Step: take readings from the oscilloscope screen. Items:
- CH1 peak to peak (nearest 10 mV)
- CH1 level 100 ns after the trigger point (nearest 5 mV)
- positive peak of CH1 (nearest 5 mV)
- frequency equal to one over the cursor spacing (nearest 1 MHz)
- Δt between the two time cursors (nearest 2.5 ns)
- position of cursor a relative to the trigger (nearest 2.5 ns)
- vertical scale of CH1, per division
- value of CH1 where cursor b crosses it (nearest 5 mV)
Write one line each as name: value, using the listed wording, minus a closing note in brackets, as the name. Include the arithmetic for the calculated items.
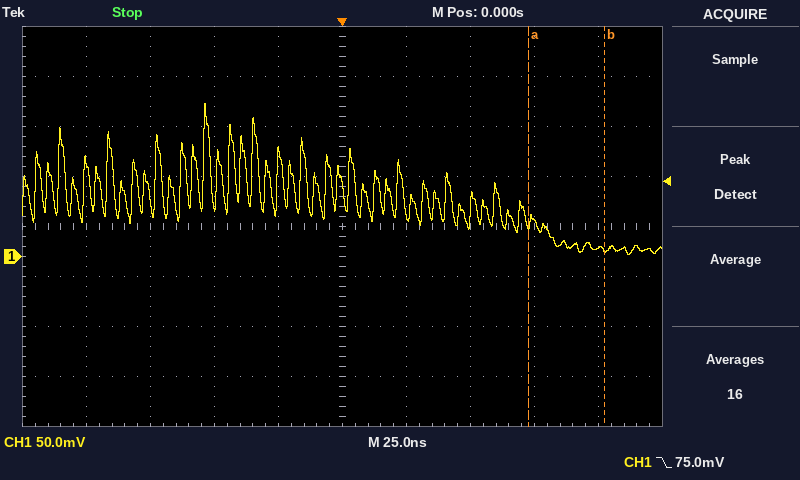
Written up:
CH1 peak to peak: 150 mV
CH1 level 100 ns after the trigger point: 10 mV
positive peak of CH1: 155 mV
frequency equal to one over the cursor spacing: 1 / 30.0 ns ≈ 33 MHz
Δt between the two time cursors: 30.0 ns
position of cursor a relative to the trigger: +72.5 ns
vertical scale of CH1, per division: 50 mV
value of CH1 where cursor b crosses it: 5 mV
